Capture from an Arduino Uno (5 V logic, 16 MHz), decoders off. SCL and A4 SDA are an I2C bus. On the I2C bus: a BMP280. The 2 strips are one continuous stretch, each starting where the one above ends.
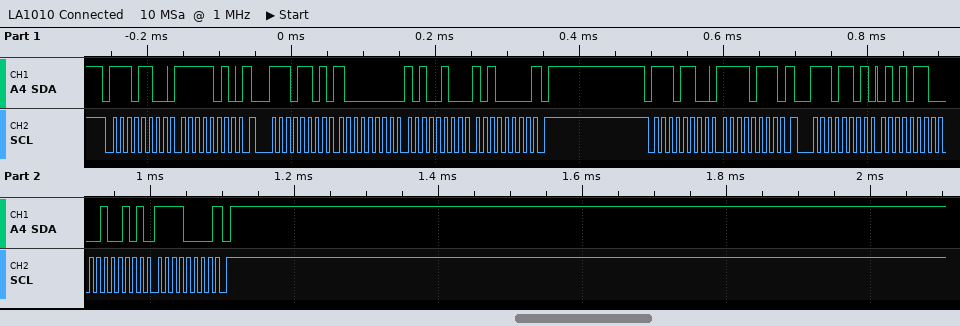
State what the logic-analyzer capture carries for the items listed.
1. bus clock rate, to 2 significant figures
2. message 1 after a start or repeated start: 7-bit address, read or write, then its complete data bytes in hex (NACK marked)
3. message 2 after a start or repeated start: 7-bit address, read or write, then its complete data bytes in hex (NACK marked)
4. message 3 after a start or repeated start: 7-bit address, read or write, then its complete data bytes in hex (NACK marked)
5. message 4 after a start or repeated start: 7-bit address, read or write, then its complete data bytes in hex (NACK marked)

100 kHz
0x76 write: FA
0x76 read: 80 A4 A0 NACK
0x76 write: F7
0x76 read: 56 25 F0 NACK
